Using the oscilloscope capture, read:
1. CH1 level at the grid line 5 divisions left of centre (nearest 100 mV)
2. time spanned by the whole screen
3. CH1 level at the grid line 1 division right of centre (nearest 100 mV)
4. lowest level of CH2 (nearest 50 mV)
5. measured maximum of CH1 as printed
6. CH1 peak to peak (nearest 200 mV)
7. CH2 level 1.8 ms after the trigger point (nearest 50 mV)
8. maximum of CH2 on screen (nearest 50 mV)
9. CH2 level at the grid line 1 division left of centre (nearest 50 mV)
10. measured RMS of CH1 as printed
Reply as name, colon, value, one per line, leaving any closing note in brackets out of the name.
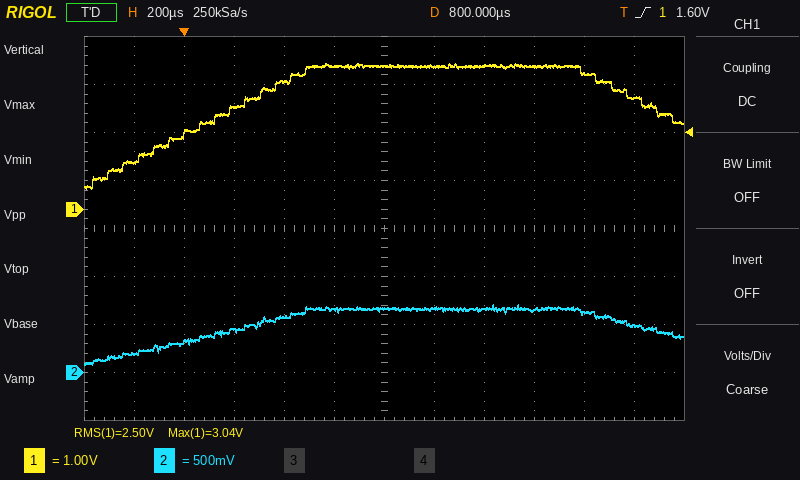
CH1 level at the grid line 5 divisions left of centre: 1.0 V
time spanned by the whole screen: 2.4 ms
CH1 level at the grid line 1 division right of centre: 3.0 V
lowest level of CH2: 100 mV
measured maximum of CH1 as printed: 3.04 V
CH1 peak to peak: 2.6 V
CH2 level 1.8 ms after the trigger point: 500 mV
maximum of CH2 on screen: 700 mV
CH2 level at the grid line 1 division left of centre: 650 mV
measured RMS of CH1 as printed: 2.50 V
